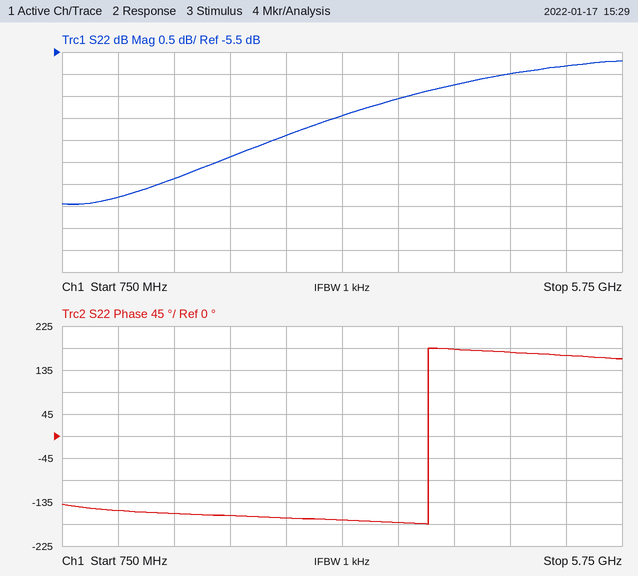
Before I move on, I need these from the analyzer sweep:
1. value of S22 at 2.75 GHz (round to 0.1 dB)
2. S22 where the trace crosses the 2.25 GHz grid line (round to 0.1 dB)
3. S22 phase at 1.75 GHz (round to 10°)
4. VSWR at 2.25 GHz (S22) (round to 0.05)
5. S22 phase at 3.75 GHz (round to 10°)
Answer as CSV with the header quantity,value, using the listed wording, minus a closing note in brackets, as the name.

quantity,value
value of S22 at 2.75 GHz,-7.4 dB
S22 where the trace crosses the 2.25 GHz grid line,-7.9 dB
S22 phase at 1.75 GHz,-160°
VSWR at 2.25 GHz (S22),2.35
S22 phase at 3.75 GHz,-180°
